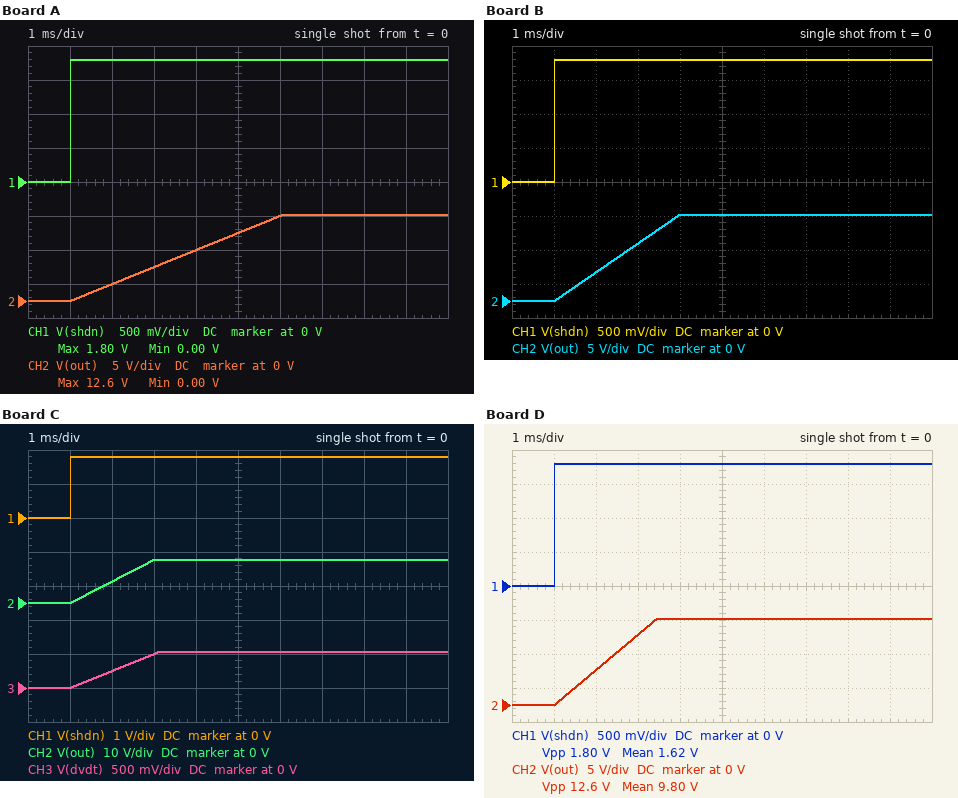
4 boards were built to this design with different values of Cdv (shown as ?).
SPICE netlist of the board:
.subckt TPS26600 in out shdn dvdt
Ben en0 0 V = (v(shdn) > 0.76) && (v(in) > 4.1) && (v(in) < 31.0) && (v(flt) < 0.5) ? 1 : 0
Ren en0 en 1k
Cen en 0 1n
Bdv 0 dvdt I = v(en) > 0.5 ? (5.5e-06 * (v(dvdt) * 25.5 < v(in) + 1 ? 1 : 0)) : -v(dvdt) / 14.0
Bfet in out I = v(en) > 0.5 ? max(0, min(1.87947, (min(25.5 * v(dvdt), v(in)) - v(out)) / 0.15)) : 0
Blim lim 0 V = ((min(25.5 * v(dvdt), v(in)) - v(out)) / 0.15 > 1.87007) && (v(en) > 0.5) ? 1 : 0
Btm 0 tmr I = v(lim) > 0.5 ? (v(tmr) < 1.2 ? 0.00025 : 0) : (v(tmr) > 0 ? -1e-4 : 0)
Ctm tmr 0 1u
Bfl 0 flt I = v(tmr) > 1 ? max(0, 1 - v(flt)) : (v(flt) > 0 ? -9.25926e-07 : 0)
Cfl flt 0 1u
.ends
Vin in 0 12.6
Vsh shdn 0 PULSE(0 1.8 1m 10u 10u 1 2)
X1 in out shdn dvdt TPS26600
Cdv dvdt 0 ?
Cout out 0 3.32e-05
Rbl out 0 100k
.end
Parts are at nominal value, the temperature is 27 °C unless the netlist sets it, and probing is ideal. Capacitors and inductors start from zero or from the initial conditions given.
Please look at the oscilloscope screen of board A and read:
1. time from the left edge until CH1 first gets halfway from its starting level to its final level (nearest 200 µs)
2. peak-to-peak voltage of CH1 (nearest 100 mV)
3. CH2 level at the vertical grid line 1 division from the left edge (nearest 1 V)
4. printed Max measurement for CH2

1.0 ms
1.8 V
0 V
12.6 V
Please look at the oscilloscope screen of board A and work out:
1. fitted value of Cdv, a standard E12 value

56 nF
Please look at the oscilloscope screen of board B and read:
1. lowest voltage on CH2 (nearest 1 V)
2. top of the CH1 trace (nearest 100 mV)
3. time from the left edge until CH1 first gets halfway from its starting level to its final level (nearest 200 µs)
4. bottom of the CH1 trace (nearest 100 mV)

0 V
1.8 V
1.0 ms
0 V
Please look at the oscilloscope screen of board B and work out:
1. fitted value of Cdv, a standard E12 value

33 nF
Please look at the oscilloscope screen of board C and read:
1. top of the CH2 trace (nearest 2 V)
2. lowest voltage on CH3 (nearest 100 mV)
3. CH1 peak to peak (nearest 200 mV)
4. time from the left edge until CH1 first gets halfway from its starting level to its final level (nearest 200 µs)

12 V
0 V
1.8 V
1.0 ms
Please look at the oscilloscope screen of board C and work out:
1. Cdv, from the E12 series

22 nF
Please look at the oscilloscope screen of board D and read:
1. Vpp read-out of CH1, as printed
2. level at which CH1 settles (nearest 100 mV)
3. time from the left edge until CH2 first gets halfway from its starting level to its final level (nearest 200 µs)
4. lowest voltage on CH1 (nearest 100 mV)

1.80 V
1.8 V
2.2 ms
0 V
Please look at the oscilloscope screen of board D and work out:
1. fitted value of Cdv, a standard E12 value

27 nF
